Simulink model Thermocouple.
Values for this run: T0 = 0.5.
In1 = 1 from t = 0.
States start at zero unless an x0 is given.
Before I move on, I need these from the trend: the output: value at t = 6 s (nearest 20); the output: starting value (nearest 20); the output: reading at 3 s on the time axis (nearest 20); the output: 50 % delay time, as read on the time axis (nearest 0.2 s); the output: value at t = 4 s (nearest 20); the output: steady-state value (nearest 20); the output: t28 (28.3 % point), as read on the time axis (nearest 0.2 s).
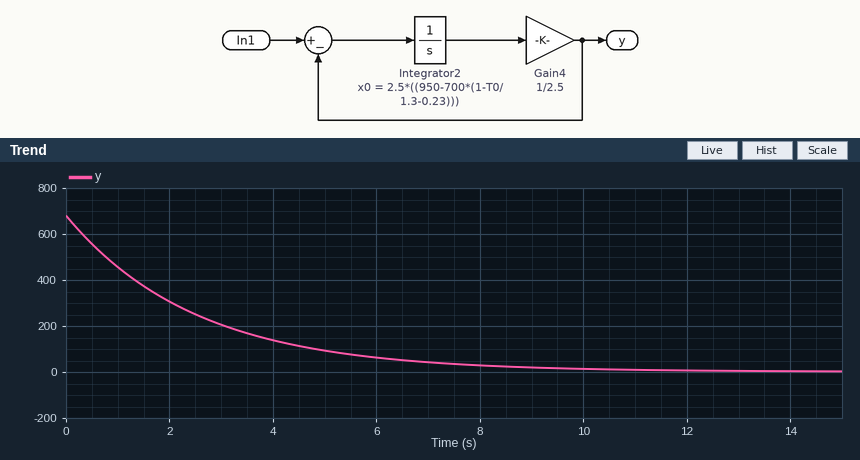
60
680
200
1.8 s
140
0
0.8 s
